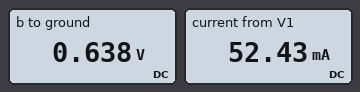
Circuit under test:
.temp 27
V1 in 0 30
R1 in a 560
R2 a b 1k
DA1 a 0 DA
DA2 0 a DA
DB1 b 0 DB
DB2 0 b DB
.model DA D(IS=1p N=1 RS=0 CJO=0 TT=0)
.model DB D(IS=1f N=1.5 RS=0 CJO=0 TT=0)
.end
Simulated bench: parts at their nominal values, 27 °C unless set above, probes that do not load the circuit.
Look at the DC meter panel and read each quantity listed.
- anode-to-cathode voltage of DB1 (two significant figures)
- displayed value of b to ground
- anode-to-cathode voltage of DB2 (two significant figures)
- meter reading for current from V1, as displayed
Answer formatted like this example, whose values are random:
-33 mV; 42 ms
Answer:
640 mV; 0.638 V; -640 mV; 52.43 mA
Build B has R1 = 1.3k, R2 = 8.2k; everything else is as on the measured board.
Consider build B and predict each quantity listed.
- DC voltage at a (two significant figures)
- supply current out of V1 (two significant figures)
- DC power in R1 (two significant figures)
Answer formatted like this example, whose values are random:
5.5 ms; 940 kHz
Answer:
620 mV; 23 mA; 660 mW
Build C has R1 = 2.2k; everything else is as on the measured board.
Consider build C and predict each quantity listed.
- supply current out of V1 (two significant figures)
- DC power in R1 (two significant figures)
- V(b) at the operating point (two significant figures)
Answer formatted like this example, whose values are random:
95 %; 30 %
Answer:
13 mA; 390 mW; 600 mV
